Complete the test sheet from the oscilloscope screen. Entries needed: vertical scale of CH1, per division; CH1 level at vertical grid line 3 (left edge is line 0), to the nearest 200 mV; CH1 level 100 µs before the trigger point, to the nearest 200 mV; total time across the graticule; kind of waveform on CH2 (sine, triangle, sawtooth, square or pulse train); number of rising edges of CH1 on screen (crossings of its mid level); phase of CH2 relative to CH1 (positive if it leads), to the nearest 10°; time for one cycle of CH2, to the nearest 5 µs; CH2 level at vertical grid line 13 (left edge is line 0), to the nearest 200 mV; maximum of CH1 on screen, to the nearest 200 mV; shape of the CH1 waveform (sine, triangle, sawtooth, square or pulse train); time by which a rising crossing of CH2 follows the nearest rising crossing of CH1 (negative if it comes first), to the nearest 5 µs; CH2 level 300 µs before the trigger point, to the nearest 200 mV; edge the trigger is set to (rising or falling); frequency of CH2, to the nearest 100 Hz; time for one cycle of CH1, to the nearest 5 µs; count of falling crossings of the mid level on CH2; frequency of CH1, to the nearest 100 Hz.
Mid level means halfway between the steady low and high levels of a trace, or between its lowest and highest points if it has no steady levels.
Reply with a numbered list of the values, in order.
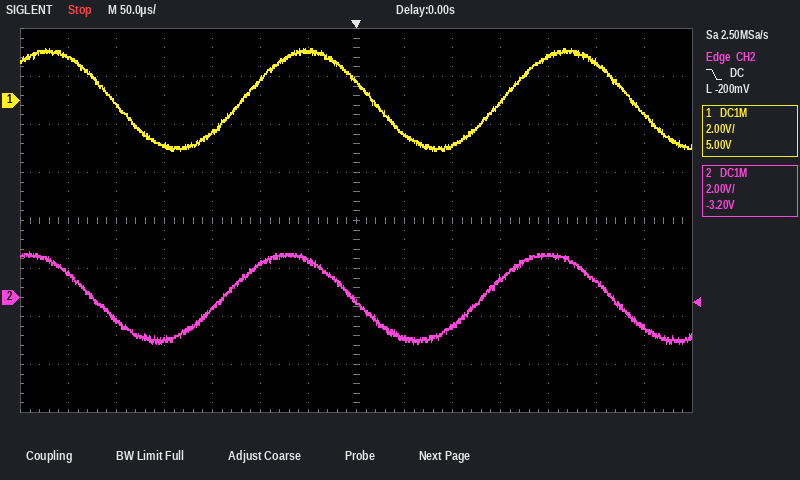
1. 2 V
2. -1.8 V
3. 800 mV
4. 700 µs
5. sine
6. 2
7. +30°
8. 270 µs
9. -1.2 V
10. 2.2 V
11. sine
12. -20 µs
13. 1.0 V
14. falling
15. 3.7 kHz
16. 270 µs
17. 3
18. 3.7 kHz
